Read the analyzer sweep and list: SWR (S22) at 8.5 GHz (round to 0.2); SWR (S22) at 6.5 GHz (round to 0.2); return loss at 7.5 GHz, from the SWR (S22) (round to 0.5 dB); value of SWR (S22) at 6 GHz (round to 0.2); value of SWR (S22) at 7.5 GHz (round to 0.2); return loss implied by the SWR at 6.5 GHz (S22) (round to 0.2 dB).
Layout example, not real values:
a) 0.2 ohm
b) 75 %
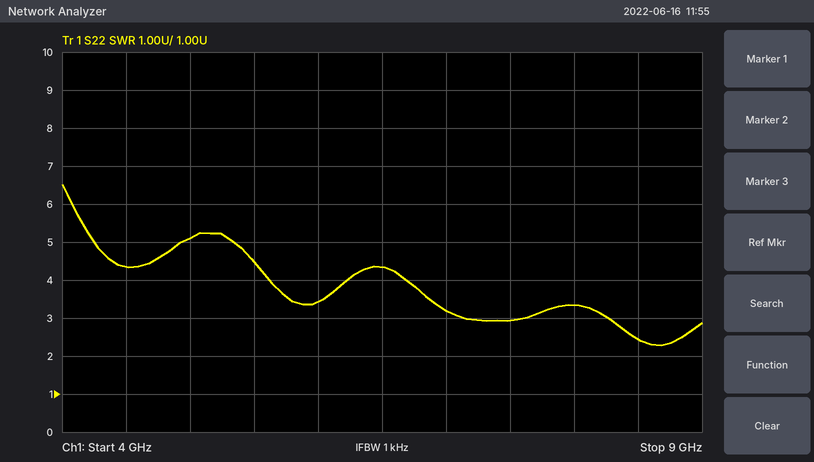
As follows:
a) 2.4
b) 4.4
c) 6.0 dB
d) 3.4
e) 3.0
f) 4.0 dB
